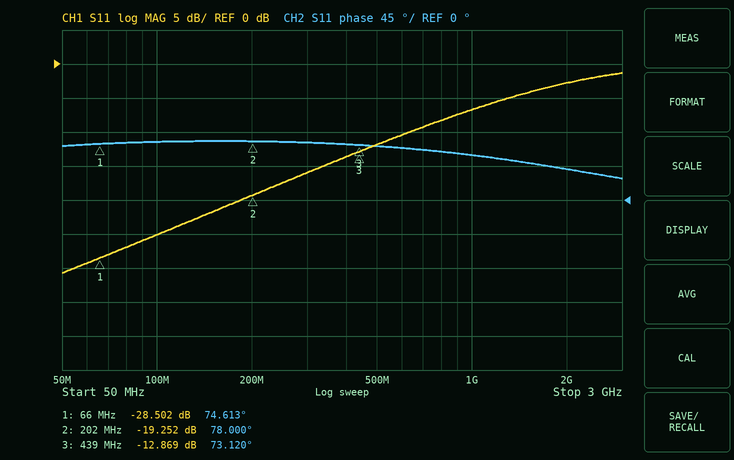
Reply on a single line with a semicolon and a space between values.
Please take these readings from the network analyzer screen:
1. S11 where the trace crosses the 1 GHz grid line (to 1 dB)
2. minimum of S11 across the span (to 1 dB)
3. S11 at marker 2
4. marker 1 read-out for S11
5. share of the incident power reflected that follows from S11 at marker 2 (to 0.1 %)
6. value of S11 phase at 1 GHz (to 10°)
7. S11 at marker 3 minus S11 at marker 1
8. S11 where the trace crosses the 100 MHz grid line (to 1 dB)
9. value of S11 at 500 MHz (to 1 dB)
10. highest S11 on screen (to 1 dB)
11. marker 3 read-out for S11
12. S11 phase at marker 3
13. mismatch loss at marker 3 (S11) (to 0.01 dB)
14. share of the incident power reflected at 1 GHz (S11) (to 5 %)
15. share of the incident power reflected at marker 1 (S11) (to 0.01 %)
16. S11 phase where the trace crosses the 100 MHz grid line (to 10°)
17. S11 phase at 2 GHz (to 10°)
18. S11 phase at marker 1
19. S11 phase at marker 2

-7 dB; -31 dB; -19.252 dB; -28.502 dB; 1.2 %; 60°; 15.633 dB; -25 dB; -12 dB; -1 dB; -12.869 dB; 73.120°; 0.23 dB; 20 %; 0.14 %; 80°; 40°; 74.613°; 78.000°
